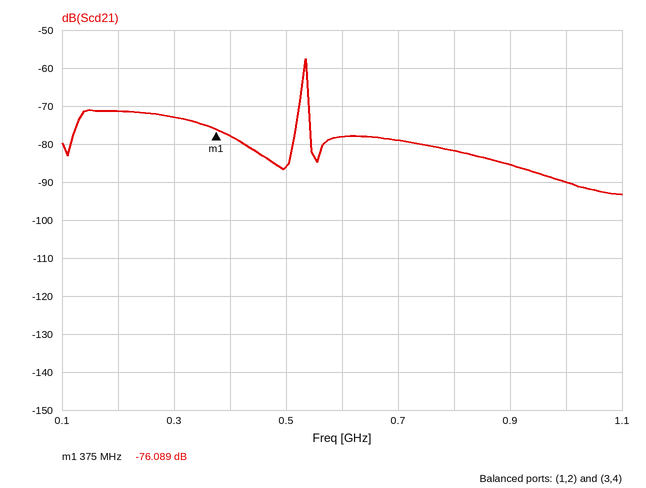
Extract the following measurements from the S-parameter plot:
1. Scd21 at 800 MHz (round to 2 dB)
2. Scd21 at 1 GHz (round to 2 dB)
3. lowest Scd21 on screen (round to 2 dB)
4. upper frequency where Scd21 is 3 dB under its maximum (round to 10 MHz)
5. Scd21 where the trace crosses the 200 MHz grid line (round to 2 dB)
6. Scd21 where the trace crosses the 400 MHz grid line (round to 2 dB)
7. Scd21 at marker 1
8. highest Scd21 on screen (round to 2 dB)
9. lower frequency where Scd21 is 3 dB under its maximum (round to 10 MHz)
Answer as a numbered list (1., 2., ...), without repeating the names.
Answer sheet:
1. -82 dB
2. -90 dB
3. -94 dB
4. 540 MHz
5. -72 dB
6. -78 dB
7. -76.089 dB
8. -58 dB
9. 530 MHz
